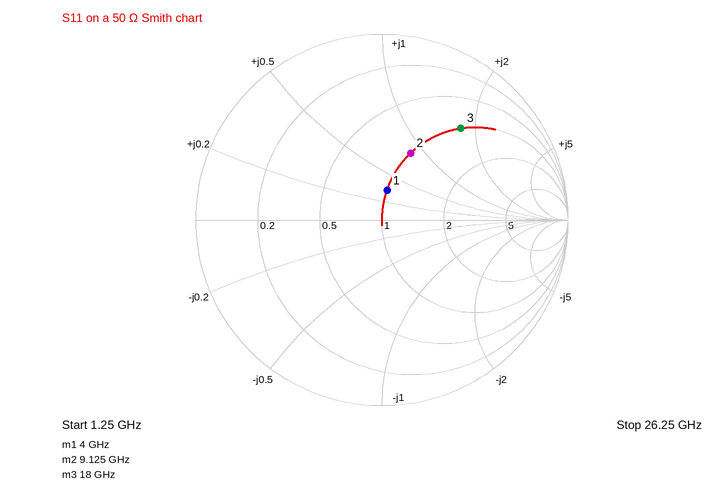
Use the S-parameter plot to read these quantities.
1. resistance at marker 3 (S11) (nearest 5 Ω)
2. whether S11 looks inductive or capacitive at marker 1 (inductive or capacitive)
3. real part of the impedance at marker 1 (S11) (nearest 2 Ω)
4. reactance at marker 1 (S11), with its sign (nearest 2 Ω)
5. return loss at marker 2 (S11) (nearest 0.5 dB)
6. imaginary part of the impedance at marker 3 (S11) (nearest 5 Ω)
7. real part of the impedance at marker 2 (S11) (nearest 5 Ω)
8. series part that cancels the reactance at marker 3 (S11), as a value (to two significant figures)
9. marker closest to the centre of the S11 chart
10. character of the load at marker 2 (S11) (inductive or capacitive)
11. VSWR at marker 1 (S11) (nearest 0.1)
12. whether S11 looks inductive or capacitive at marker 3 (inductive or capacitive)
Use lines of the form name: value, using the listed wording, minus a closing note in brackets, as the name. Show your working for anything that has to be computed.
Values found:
resistance at marker 3 (S11): 50 Ω
whether S11 looks inductive or capacitive at marker 1: inductive
real part of the impedance at marker 1 (S11): 50 Ω
reactance at marker 1 (S11), with its sign: +16 Ω
return loss at marker 2 (S11): 8.0 dB
imaginary part of the impedance at marker 3 (S11): +85 Ω
real part of the impedance at marker 2 (S11): 50 Ω
series part that cancels the reactance at marker 3 (S11), as a value: C = 1/(2π × 18 GHz × 85 Ω) ≈ 104 fF, so 100 fF to two significant figures
marker closest to the centre of the S11 chart: marker 1
character of the load at marker 2 (S11): inductive
VSWR at marker 1 (S11): 1.4
whether S11 looks inductive or capacitive at marker 3: inductive
